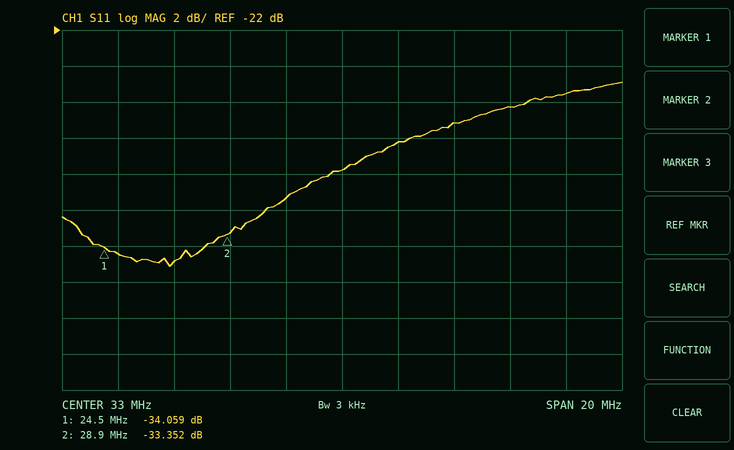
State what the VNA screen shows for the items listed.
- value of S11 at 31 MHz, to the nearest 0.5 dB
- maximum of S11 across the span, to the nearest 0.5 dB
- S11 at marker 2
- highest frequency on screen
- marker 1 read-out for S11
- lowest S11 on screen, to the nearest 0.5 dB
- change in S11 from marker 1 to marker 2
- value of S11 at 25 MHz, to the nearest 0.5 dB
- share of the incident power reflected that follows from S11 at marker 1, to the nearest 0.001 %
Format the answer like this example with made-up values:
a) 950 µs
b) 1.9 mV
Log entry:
a) -31.5 dB
b) -25.0 dB
c) -33.352 dB
d) 43 MHz
e) -34.059 dB
f) -35.0 dB
g) 0.707 dB
h) -34.5 dB
i) 0.039 %
